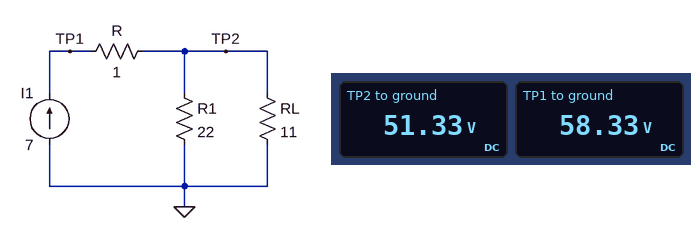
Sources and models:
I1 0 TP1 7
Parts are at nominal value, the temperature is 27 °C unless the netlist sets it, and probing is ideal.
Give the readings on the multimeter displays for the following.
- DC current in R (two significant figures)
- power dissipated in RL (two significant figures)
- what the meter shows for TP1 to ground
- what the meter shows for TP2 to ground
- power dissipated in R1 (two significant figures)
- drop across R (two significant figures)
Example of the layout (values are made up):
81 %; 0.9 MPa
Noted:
7.0 A; 240 W; 58.33 V; 51.33 V; 120 W; 7.0 V
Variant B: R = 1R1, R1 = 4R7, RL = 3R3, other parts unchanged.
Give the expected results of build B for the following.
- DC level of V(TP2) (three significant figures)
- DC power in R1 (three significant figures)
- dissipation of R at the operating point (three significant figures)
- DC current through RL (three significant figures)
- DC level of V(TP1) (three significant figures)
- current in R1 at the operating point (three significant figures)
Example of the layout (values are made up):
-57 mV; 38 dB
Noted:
13.6 V; 39.2 W; 53.9 W; 4.11 A; 21.3 V; 2.89 A
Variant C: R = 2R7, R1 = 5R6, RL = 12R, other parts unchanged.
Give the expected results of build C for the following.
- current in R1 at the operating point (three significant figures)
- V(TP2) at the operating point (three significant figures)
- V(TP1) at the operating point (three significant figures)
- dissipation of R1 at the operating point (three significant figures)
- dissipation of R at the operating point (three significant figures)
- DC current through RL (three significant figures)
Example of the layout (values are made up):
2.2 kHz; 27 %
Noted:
4.77 A; 26.7 V; 45.6 V; 128 W; 132 W; 2.23 A
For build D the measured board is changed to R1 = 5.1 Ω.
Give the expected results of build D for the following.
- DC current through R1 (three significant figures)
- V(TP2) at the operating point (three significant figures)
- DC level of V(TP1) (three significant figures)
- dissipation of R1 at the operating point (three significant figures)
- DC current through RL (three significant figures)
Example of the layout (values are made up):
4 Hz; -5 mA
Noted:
4.78 A; 24.4 V; 31.4 V; 117 W; 2.22 A
